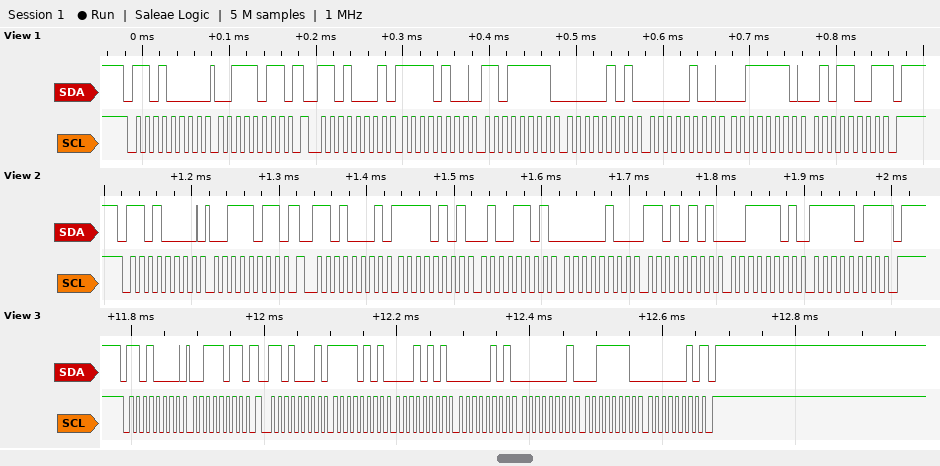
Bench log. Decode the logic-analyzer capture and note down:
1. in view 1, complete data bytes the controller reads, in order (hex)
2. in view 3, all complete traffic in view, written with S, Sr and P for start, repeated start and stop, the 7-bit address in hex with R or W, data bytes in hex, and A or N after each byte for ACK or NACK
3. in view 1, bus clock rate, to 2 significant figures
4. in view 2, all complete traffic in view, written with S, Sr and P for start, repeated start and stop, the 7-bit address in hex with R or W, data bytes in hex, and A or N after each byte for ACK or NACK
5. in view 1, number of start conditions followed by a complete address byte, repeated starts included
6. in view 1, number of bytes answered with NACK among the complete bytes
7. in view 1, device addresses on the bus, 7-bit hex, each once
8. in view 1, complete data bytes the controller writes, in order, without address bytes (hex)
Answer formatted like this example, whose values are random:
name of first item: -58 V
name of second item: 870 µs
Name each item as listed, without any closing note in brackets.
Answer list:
in view 1, complete data bytes the controller reads, in order: F4 DF 05 04 3E 59
in view 3, all complete traffic in view, written with S, Sr and P for start, repeated start and stop, the 7-bit address in hex with R or W, data bytes in hex, and A or N after each byte for ACK or NACK: S 68W A 3B A Sr 68R A F5 A 15 A 05 A 01 A 3E A 02 N P
in view 1, bus clock rate, to 2 significant figures: 100 kHz
in view 2, all complete traffic in view, written with S, Sr and P for start, repeated start and stop, the 7-bit address in hex with R or W, data bytes in hex, and A or N after each byte for ACK or NACK: S 68W A 3B A Sr 68R A F5 A 4D A 04 A D5 A 3D A FB N P
in view 1, number of start conditions followed by a complete address byte, repeated starts included: 2
in view 1, number of bytes answered with NACK among the complete bytes: 1
in view 1, device addresses on the bus, 7-bit hex, each once: 0x68
in view 1, complete data bytes the controller writes, in order, without address bytes: 3B
